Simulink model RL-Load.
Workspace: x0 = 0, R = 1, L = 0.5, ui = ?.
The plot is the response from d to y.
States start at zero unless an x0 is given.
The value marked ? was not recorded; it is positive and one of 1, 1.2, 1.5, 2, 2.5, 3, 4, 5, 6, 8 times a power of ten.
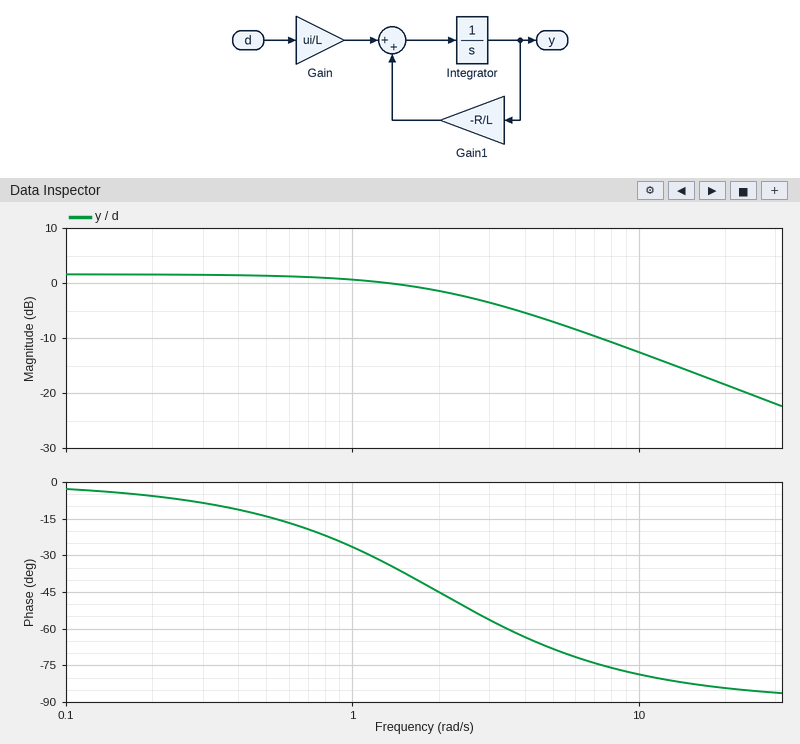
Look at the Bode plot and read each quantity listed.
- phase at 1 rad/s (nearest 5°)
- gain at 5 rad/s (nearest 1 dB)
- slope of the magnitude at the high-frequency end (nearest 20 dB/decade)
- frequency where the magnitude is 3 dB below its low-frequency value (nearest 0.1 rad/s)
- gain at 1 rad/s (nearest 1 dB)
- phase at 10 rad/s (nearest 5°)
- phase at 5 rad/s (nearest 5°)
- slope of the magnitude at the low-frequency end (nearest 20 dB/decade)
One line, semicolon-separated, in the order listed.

-25°; -7 dB; -20 dB/decade; 2.0 rad/s; 1 dB; -80°; -70°; 0 dB/decade
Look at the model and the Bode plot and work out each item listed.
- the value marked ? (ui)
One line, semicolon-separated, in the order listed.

1.2
